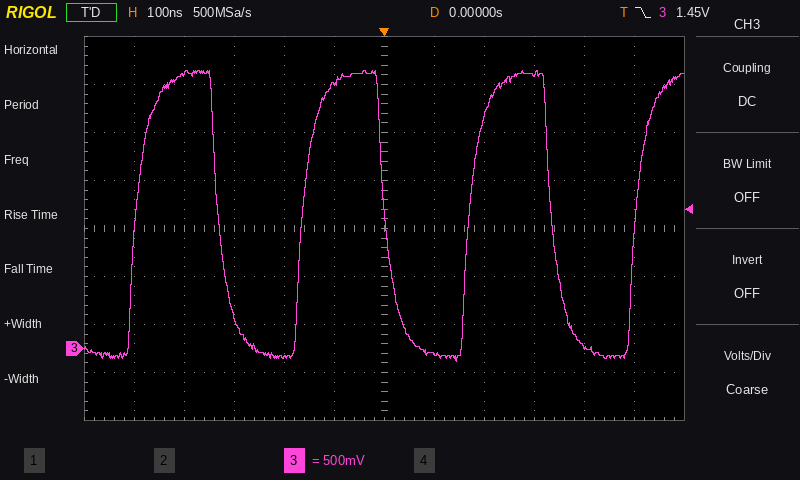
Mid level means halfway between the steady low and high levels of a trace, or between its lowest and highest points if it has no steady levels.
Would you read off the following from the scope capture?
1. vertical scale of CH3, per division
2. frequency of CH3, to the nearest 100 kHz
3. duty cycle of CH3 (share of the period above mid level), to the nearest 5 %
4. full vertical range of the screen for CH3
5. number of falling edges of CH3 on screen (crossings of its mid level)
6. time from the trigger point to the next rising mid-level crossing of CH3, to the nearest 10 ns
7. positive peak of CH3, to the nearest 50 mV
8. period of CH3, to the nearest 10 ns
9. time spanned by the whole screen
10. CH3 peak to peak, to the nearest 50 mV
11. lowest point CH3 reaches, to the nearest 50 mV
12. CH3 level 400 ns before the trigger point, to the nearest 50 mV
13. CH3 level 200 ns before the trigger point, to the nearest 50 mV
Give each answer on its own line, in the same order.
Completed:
500 mV
3.0 MHz
50 %
4 V
3
170 ns
2.90 V
330 ns
1.2 µs
3.05 V
-150 mV
2.85 V
-100 mV
